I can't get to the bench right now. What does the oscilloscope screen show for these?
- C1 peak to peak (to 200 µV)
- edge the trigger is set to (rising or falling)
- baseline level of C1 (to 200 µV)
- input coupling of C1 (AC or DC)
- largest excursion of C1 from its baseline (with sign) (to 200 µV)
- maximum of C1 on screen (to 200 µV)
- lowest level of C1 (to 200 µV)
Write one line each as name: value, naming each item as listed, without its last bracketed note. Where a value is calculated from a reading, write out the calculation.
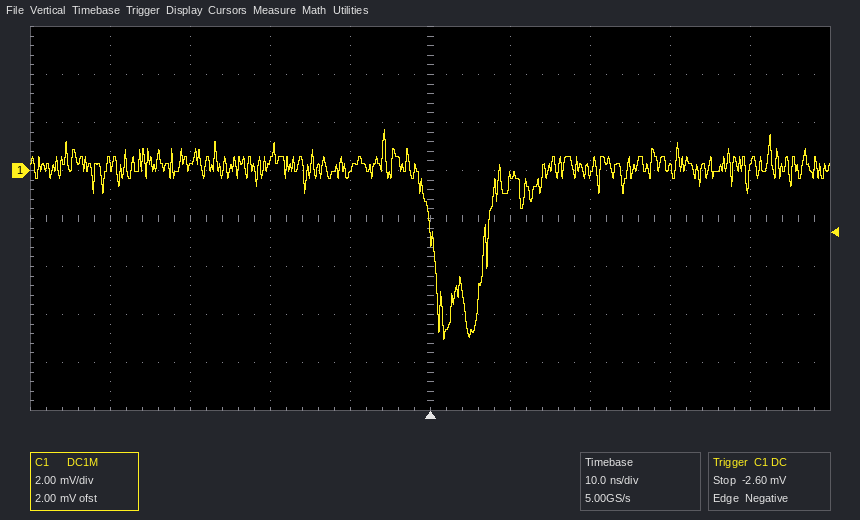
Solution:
C1 peak to peak: 1.8 mV − (-7.0 mV) = 8.8 mV
edge the trigger is set to: falling
baseline level of C1: 200 µV
input coupling of C1: DC
largest excursion of C1 from its baseline (with sign): -7.0 mV − (200 µV) = -7.2 mV
maximum of C1 on screen: 1.8 mV
lowest level of C1: -7.0 mV
